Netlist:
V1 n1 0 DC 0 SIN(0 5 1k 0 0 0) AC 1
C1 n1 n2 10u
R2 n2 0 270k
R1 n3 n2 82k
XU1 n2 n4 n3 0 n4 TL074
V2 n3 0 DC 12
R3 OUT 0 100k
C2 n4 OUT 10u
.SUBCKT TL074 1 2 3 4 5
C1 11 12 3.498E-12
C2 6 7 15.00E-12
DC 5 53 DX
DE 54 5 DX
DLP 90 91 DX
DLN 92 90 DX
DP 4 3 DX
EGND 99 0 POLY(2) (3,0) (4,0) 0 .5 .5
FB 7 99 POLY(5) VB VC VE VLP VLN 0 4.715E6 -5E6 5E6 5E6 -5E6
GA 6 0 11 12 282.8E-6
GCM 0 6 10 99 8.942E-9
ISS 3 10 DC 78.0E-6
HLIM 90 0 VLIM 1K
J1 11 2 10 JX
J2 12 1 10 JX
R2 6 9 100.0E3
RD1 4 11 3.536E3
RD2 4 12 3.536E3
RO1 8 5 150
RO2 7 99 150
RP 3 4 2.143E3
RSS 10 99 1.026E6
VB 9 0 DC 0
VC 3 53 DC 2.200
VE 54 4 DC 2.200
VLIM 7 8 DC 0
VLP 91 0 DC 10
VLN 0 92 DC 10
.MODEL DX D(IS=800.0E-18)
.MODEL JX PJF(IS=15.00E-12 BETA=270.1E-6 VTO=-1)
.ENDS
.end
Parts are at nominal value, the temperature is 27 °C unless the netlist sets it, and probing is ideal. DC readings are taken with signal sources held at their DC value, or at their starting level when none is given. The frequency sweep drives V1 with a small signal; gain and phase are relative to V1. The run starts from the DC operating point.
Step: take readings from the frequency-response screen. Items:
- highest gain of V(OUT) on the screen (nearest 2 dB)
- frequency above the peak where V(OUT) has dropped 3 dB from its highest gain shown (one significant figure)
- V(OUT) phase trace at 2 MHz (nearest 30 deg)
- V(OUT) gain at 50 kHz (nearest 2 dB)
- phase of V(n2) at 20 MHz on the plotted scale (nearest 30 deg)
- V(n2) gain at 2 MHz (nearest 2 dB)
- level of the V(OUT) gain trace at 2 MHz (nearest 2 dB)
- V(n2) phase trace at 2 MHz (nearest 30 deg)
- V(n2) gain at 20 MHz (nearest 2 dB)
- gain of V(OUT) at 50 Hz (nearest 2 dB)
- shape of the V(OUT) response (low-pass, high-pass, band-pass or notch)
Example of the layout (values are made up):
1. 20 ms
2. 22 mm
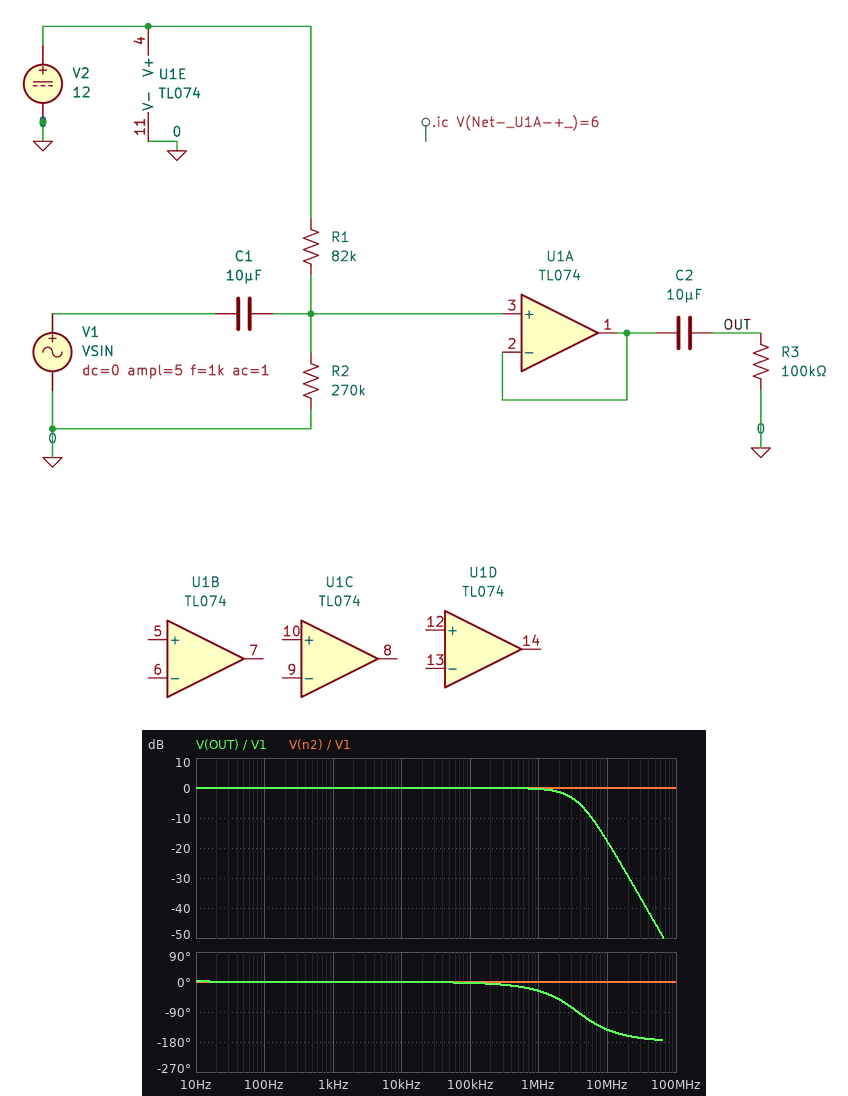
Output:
1. 0 dB
2. 3 MHz
3. -60 deg
4. 0 dB
5. 0 deg
6. 0 dB
7. -2 dB
8. 0 deg
9. 0 dB
10. 0 dB
11. low-pass
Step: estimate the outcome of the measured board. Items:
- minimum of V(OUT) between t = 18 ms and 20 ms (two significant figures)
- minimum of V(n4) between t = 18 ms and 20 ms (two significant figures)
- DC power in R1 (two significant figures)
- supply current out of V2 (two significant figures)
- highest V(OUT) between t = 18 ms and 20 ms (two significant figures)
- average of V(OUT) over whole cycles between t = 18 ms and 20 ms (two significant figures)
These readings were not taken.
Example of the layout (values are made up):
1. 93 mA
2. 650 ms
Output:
1. -5.0 V
2. 4.2 V
3. 95 µW
4. 5.7 mA
5. 1.3 V
6. -1.0 V
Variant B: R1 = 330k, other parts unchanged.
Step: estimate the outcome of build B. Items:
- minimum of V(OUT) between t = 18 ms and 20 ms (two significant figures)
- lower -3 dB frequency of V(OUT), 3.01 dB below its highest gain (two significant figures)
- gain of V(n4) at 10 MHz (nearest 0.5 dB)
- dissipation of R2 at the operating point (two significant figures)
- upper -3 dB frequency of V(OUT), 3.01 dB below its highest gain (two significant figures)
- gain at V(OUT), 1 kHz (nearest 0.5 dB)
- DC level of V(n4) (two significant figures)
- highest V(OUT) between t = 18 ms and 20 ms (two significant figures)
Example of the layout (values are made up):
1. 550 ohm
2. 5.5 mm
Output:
1. -3.9 V
2. 210 mHz
3. -17.5 dB
4. 110 µW
5. 3.0 MHz
6. 0 dB
7. 5.4 V
8. 5.0 V
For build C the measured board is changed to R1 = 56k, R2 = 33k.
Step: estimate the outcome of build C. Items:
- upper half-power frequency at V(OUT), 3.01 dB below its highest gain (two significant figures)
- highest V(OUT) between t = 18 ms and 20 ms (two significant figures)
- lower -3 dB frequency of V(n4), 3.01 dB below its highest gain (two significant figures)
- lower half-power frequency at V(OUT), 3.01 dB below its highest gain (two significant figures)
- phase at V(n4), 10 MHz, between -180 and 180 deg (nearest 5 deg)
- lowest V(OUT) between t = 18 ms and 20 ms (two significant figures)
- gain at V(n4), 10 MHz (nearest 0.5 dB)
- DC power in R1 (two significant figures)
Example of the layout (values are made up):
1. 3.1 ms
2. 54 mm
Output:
1. 3.0 MHz
2. 6.0 V
3. 770 mHz
4. 800 mHz
5. -145 deg
6. -2.9 V
7. -17.5 dB
8. 1.0 mW
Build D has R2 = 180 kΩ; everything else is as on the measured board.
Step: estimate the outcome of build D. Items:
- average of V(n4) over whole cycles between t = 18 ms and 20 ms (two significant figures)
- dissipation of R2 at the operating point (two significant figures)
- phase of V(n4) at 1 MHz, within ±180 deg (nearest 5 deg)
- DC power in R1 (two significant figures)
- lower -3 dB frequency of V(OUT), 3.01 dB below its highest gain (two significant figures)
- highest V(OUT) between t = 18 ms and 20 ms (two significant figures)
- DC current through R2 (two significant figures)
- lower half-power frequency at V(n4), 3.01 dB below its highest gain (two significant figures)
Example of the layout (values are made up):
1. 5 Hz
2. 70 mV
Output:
1. 7.6 V
2. 380 µW
3. -25 deg
4. 170 µW
5. 350 mHz
6. 2.2 V
7. 46 µA
8. 280 mHz
